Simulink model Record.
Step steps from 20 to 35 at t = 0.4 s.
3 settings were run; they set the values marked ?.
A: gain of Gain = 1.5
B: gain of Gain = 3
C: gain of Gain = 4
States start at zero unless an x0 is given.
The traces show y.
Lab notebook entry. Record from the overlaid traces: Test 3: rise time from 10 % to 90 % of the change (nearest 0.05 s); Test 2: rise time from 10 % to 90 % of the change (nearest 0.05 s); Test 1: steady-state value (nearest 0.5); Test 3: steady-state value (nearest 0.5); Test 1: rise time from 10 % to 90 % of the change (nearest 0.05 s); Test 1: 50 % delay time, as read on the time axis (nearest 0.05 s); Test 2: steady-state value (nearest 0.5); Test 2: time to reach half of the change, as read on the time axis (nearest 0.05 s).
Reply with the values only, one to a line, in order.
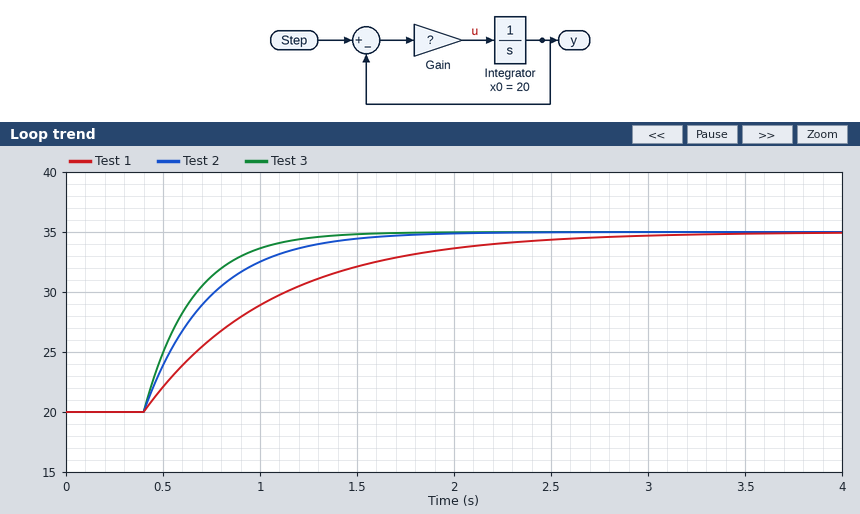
0.55 s
0.75 s
35.0
35.0
1.45 s
0.85 s
35.0
0.65 s
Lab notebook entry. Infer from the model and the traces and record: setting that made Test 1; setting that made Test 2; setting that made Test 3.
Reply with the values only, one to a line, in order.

A
B
C
